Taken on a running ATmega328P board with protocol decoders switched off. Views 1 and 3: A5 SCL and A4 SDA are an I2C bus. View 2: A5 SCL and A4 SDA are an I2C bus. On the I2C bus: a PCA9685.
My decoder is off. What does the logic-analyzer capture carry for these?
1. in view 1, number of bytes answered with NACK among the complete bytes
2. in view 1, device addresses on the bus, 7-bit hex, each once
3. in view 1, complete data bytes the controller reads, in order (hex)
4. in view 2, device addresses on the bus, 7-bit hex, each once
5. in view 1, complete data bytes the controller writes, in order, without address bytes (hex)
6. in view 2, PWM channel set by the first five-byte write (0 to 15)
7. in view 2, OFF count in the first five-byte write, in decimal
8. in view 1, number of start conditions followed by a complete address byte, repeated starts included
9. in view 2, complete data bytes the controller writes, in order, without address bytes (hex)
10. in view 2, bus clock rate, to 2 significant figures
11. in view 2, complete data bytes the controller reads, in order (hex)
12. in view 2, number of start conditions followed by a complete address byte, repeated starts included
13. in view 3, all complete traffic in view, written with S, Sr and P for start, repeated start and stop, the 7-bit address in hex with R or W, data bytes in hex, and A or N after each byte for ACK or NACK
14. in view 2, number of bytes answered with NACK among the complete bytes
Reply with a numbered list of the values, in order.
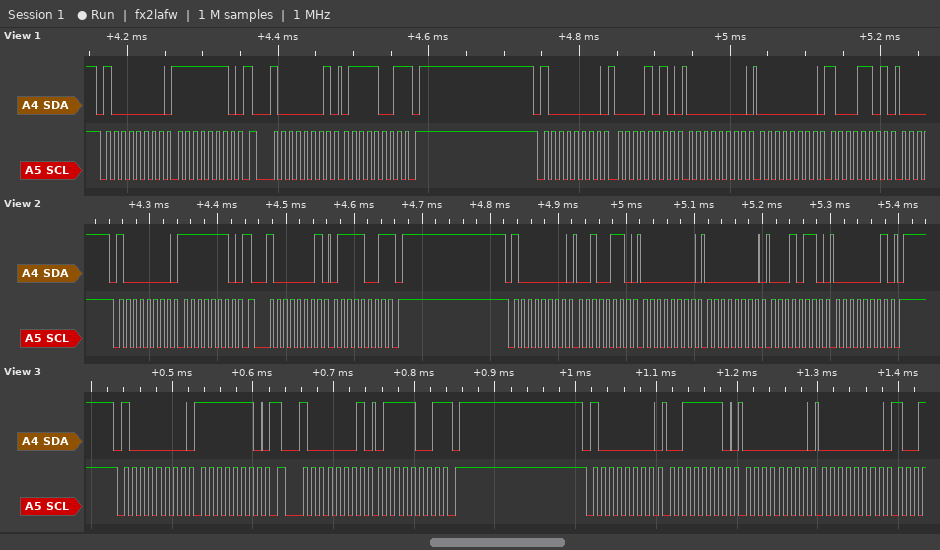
1. 1
2. 0x40
3. 79
4. 0x40
5. FE 0A 00 00 8D
6. 8
7. 278
8. 3
9. FE 26 00 00 16 01
10. 100 kHz
11. 79
12. 3
13. S 40W A FE A Sr 40R A 79 N P S 40W A 3E A 00 A 00 A
14. 1
